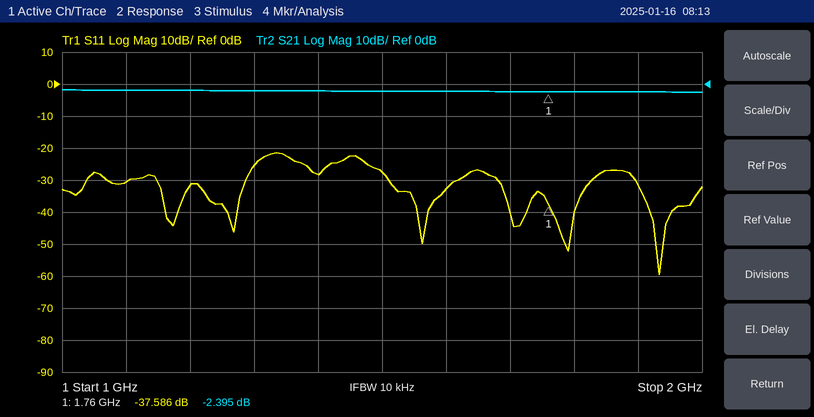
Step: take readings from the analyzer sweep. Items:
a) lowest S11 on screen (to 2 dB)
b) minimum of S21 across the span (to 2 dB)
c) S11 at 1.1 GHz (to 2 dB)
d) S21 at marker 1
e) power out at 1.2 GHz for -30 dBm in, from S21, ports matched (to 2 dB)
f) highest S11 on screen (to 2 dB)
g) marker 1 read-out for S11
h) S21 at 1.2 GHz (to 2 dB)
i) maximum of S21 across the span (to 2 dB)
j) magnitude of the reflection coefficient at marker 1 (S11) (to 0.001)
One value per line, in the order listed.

-60 dB
-2 dB
-30 dB
-2.395 dB
-32 dBm
-22 dB
-37.586 dB
-2 dB
-2 dB
0.013
